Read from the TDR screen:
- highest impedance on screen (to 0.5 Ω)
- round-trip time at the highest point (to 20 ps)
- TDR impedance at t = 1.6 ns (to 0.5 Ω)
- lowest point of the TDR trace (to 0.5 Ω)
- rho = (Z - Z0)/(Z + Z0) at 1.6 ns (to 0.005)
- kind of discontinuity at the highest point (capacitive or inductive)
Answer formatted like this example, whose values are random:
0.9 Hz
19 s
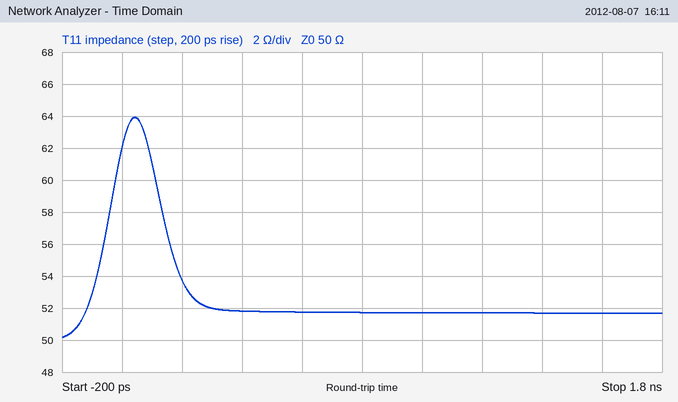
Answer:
64.0 Ω
40 ps
51.5 Ω
50.0 Ω
+0.015
inductive
